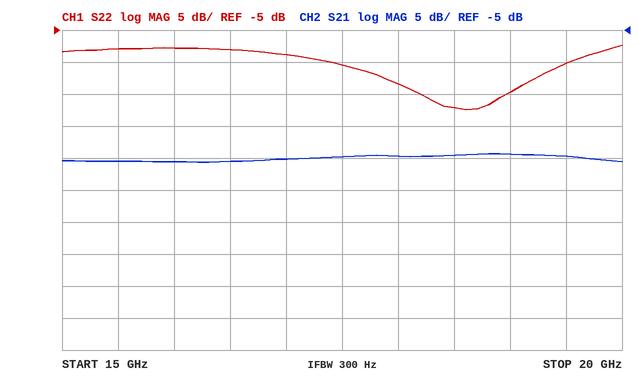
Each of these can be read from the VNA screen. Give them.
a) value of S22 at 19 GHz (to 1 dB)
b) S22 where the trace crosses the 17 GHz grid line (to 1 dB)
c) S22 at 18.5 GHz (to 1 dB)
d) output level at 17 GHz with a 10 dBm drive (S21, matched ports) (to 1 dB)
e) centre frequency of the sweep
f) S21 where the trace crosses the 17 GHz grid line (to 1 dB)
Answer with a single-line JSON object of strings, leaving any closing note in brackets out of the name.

{"value of S22 at 19 GHz": "-15 dB", "S22 where the trace crosses the 17 GHz grid line": "-9 dB", "S22 at 18.5 GHz": "-17 dB", "output level at 17 GHz with a 10 dBm drive (S21, matched ports)": "-15 dBm", "centre frequency of the sweep": "17.5 GHz", "S21 where the trace crosses the 17 GHz grid line": "-25 dB"}
